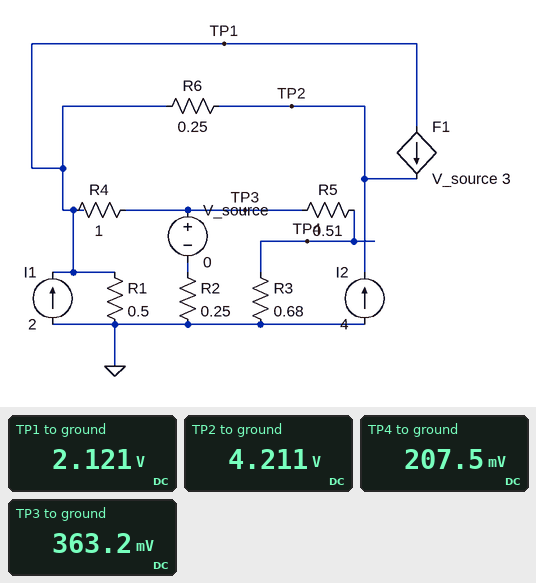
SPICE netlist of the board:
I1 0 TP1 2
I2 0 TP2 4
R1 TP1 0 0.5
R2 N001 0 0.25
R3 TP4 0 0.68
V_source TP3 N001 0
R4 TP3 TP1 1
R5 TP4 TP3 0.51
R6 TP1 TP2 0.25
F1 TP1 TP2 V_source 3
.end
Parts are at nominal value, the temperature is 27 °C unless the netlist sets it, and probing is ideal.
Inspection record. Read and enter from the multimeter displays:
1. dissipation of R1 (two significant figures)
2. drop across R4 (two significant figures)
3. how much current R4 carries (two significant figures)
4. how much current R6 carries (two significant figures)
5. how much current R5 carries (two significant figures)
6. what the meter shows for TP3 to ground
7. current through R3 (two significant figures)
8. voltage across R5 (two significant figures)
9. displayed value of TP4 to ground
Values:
9.0 W
1.8 V
1.8 A
8.4 A
310 mA
363.2 mV
310 mA
160 mV
207.5 mV
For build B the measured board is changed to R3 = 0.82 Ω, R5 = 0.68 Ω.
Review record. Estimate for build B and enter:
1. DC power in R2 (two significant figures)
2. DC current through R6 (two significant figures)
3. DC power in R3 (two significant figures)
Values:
560 mW
8.5 A
51 mW
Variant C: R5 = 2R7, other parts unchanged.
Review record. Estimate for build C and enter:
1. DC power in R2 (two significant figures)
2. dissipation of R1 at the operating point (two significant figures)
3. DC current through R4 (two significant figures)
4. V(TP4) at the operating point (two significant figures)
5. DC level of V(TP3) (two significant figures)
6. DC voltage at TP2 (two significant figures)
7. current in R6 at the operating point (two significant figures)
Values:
650 mW
9.1 W
1.7 A
81 mV
400 mV
4.3 V
8.8 A
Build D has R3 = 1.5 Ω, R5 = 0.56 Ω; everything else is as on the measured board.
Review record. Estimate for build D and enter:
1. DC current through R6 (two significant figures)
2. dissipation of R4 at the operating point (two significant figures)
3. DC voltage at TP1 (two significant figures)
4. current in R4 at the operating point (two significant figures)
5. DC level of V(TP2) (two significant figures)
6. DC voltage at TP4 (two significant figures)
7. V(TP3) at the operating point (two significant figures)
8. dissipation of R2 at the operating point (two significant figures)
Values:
8.7 A
3.0 W
2.1 V
1.7 A
4.3 V
280 mV
390 mV
600 mW
